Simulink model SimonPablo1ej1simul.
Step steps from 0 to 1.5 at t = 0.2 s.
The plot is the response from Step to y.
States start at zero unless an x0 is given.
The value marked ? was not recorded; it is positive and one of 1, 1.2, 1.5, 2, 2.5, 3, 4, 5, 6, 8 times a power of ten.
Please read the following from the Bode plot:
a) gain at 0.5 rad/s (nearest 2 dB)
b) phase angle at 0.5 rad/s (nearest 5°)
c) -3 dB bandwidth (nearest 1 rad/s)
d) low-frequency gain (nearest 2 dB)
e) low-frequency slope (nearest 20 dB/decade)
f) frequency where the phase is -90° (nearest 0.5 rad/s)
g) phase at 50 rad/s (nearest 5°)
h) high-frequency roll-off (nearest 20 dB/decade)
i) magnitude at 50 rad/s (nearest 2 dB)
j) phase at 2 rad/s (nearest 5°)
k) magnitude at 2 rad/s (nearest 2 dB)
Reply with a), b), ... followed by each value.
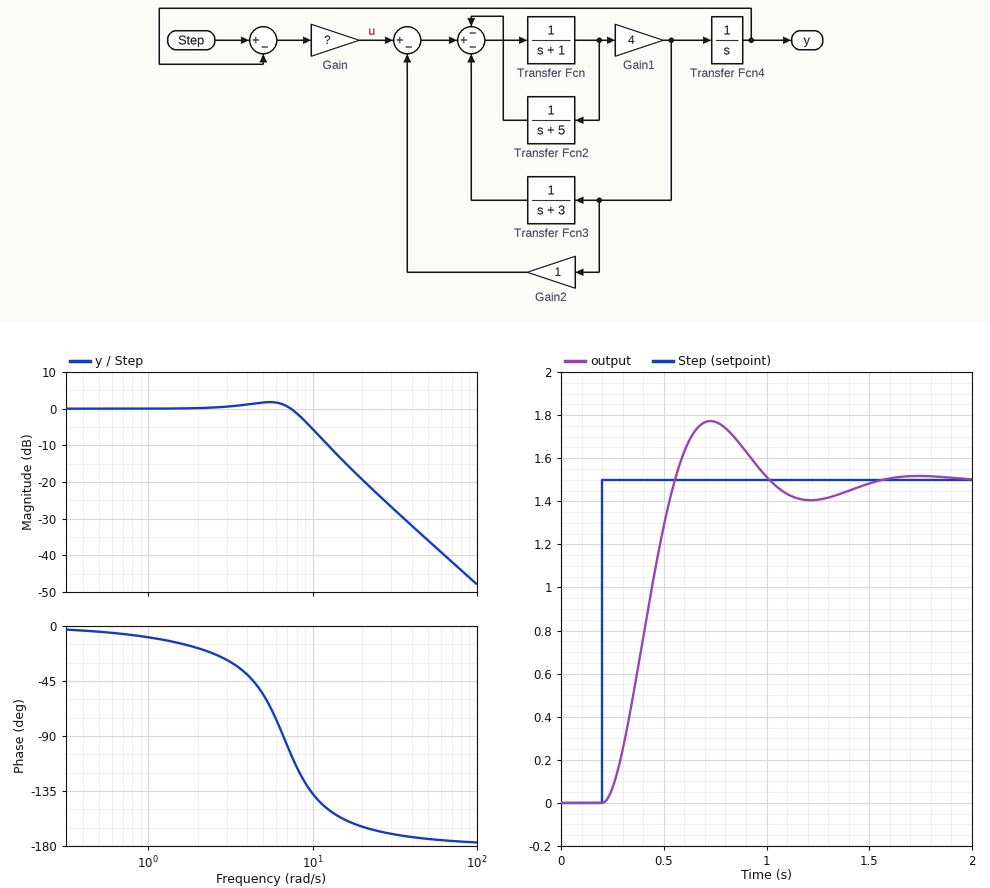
a) 0 dB
b) -5°
c) 9 rad/s
d) 0 dB
e) 0 dB/decade
f) 6.5 rad/s
g) -175°
h) -40 dB/decade
i) -36 dB
j) -20°
k) 0 dB
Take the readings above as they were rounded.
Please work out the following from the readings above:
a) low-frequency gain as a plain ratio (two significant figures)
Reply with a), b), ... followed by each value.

a) 1.0
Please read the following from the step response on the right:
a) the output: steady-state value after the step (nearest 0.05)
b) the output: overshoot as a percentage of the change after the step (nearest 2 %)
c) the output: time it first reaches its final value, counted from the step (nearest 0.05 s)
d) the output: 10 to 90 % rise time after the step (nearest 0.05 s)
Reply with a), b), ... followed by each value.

a) 1.50
b) 18 %
c) 0.35 s
d) 0.25 s
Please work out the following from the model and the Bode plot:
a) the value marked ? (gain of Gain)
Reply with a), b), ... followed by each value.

a) 10
